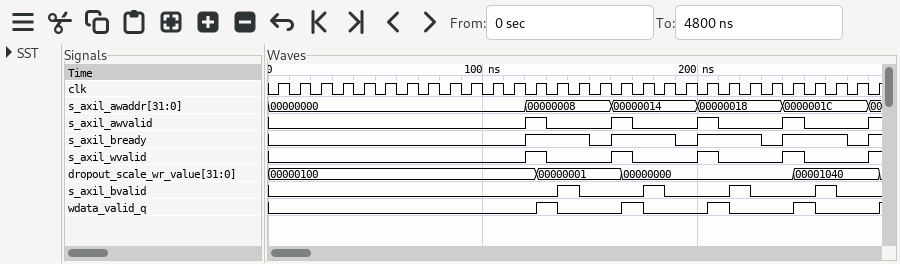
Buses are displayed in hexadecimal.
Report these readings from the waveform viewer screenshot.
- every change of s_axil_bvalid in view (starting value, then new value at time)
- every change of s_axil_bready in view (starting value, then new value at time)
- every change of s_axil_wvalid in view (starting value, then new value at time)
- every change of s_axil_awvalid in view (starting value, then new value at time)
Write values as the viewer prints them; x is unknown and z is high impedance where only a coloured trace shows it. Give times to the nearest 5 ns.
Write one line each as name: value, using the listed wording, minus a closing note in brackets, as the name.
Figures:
every change of s_axil_bvalid in view: 0, 1 at 135 ns, 0 at 145 ns, 1 at 175 ns, 0 at 185 ns, 1 at 215 ns, 0 at 225 ns, 1 at 255 ns, 0 at 265 ns
every change of s_axil_bready in view: 0, 1 at 120 ns, 0 at 150 ns, 1 at 160 ns, 0 at 190 ns, 1 at 200 ns, 0 at 230 ns, 1 at 240 ns, 0 at 270 ns, 1 at 280 ns
every change of s_axil_wvalid in view: 0, 1 at 120 ns, 0 at 130 ns, 1 at 160 ns, 0 at 170 ns, 1 at 200 ns, 0 at 210 ns, 1 at 240 ns, 0 at 250 ns, 1 at 280 ns
every change of s_axil_awvalid in view: 0, 1 at 120 ns, 0 at 130 ns, 1 at 160 ns, 0 at 170 ns, 1 at 200 ns, 0 at 210 ns, 1 at 240 ns, 0 at 250 ns, 1 at 280 ns
